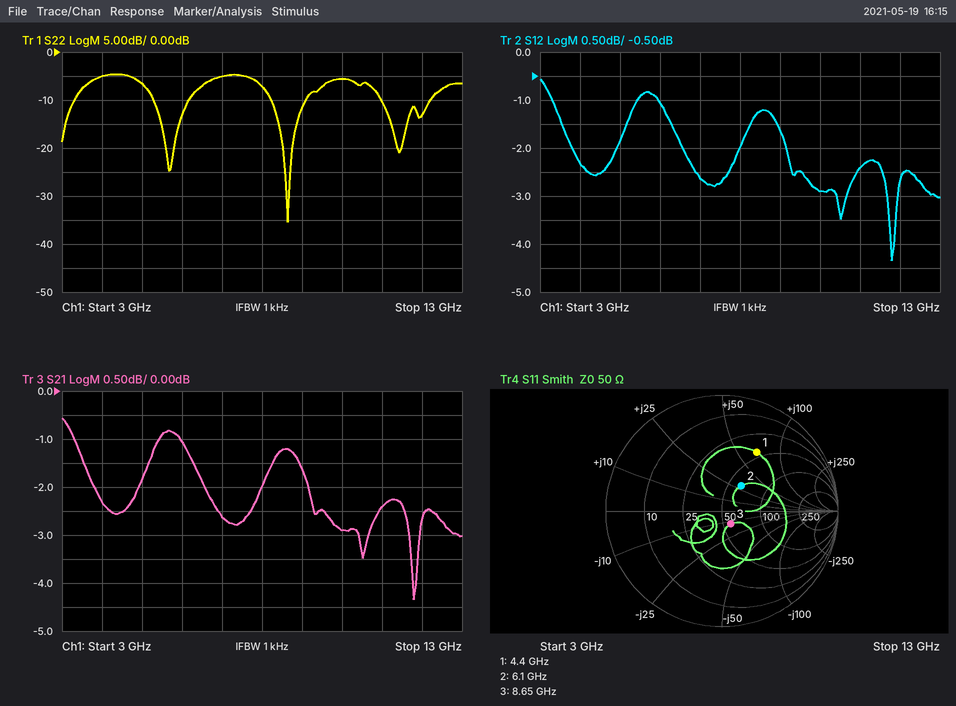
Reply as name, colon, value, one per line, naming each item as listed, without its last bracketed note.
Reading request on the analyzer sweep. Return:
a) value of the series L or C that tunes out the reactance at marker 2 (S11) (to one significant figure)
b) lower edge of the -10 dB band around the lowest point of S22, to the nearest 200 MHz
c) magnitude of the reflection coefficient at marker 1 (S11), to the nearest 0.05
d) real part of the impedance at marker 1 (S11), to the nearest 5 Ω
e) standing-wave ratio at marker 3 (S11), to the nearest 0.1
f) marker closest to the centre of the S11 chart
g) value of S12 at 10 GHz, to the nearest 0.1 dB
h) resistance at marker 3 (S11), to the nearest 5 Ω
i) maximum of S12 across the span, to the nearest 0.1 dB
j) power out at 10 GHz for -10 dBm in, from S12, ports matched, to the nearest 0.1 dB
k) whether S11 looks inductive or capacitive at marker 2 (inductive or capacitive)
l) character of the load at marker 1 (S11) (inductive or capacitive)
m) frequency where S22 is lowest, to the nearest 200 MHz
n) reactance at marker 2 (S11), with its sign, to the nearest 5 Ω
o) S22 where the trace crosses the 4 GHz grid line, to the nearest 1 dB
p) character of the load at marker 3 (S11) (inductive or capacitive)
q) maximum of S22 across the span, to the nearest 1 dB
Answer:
value of the series L or C that tunes out the reactance at marker 2 (S11): 900 fF
lower edge of the -10 dB band around the lowest point of S22, to the nearest 200 MHz: 8.2 GHz
magnitude of the reflection coefficient at marker 1 (S11), to the nearest 0.05: 0.60
real part of the impedance at marker 1 (S11), to the nearest 5 Ω: 45 Ω
standing-wave ratio at marker 3 (S11), to the nearest 0.1: 1.3
marker closest to the centre of the S11 chart: marker 3
value of S12 at 10 GHz, to the nearest 0.1 dB: -2.9 dB
resistance at marker 3 (S11), to the nearest 5 Ω: 55 Ω
maximum of S12 across the span, to the nearest 0.1 dB: -0.6 dB
power out at 10 GHz for -10 dBm in, from S12, ports matched, to the nearest 0.1 dB: -12.9 dBm
whether S11 looks inductive or capacitive at marker 2: inductive
character of the load at marker 1 (S11): inductive
frequency where S22 is lowest, to the nearest 200 MHz: 8.6 GHz
reactance at marker 2 (S11), with its sign, to the nearest 5 Ω: +30 Ω
S22 where the trace crosses the 4 GHz grid line, to the nearest 1 dB: -5 dB
character of the load at marker 3 (S11): capacitive
maximum of S22 across the span, to the nearest 1 dB: -5 dB
